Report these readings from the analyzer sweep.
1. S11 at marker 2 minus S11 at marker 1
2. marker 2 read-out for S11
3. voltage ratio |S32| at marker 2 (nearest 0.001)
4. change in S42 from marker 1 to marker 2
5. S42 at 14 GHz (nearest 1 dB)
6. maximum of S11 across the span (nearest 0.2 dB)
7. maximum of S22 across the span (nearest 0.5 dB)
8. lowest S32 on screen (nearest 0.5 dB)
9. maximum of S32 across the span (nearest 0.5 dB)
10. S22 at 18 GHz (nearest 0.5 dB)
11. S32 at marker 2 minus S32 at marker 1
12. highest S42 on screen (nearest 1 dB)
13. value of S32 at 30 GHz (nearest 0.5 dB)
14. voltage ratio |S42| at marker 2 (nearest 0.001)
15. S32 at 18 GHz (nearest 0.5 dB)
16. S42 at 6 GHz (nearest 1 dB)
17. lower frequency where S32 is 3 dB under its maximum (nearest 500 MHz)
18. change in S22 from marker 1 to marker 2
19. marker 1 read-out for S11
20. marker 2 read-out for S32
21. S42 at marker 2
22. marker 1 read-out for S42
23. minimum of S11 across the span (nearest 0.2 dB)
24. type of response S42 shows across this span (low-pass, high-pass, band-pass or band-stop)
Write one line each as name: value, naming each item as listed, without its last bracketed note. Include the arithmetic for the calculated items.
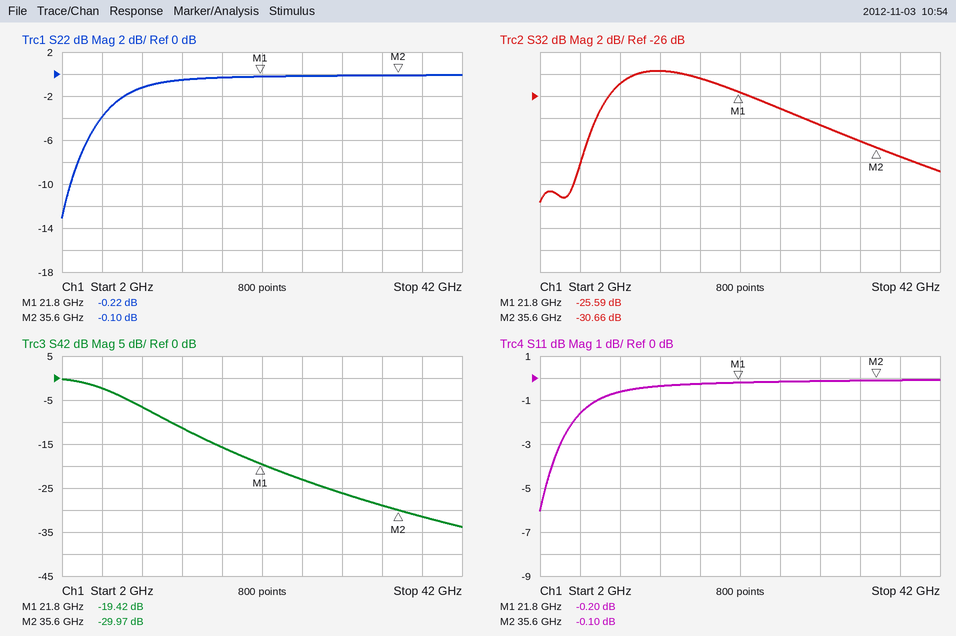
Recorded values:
S11 at marker 2 minus S11 at marker 1: -0.1 − (-0.2) = 0.10 dB
marker 2 read-out for S11: -0.10 dB
voltage ratio |S32| at marker 2: 10^(-30.66/20) ≈ 0.029
change in S42 from marker 1 to marker 2: -29.97 − (-19.42) = -10.55 dB
S42 at 14 GHz: -11 dB
maximum of S11 across the span: 0.0 dB
maximum of S22 across the span: 0.0 dB
lowest S32 on screen: -35.5 dB
maximum of S32 across the span: -23.5 dB
S22 at 18 GHz: -0.5 dB
S32 at marker 2 minus S32 at marker 1: -30.66 − (-25.59) = -5.07 dB
highest S42 on screen: 0 dB
value of S32 at 30 GHz: -28.5 dB
voltage ratio |S42| at marker 2: 10^(-29.97/20) ≈ 0.032
S32 at 18 GHz: -24.5 dB
S42 at 6 GHz: -2 dB
lower frequency where S32 is 3 dB under its maximum: 8.5 GHz
change in S22 from marker 1 to marker 2: -0.1 − (-0.22) = 0.12 dB
marker 1 read-out for S11: -0.20 dB
marker 2 read-out for S32: -30.66 dB
S42 at marker 2: -29.97 dB
marker 1 read-out for S42: -19.42 dB
minimum of S11 across the span: -6.0 dB
type of response S42 shows across this span: low-pass
